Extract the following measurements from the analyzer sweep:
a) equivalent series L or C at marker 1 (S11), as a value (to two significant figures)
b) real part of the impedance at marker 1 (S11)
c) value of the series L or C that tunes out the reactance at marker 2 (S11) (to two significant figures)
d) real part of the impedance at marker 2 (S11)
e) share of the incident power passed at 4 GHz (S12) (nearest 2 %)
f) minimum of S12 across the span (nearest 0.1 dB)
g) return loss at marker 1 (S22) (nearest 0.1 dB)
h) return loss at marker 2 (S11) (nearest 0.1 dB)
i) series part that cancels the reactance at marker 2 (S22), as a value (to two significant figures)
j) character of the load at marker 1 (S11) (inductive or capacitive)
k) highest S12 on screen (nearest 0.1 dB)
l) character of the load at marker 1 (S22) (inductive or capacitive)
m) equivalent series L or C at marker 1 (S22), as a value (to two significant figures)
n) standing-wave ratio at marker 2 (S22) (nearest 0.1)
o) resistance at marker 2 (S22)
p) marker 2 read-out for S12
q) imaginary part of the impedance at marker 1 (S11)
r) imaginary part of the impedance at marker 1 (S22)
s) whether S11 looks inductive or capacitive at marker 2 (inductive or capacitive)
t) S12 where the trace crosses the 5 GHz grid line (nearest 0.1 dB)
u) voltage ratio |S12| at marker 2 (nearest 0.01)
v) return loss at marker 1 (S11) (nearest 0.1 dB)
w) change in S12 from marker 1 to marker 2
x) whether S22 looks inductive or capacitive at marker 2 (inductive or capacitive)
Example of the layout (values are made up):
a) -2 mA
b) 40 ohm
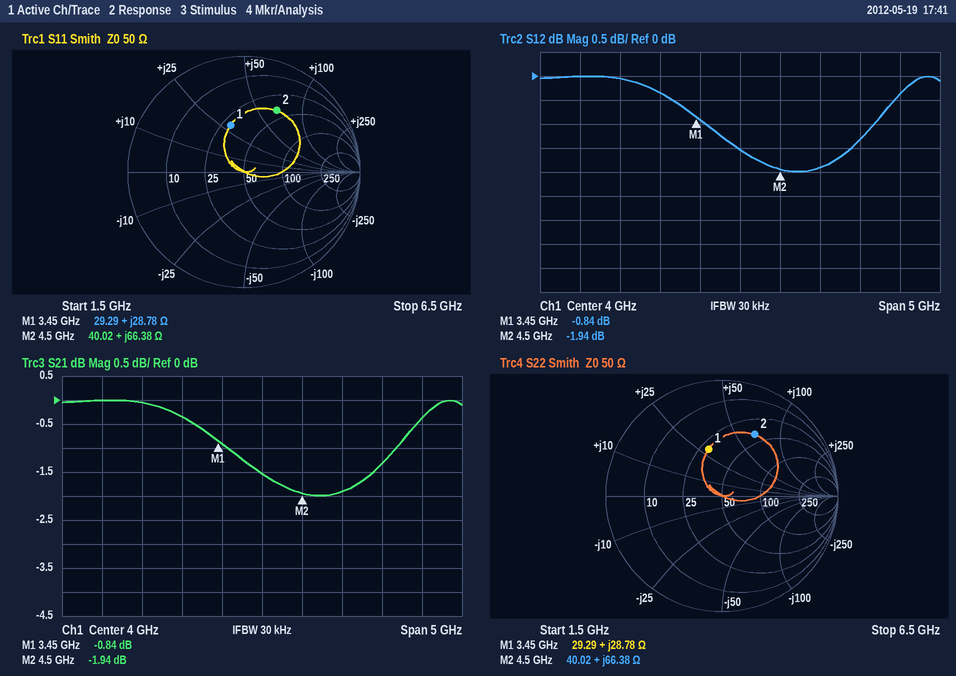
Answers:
a) 1.3 nH
b) 29.29 Ω
c) 530 fF
d) 40.02 Ω
e) 70 %
f) -2.0 dB
g) 7.5 dB
h) 4.4 dB
i) 530 fF
j) inductive
k) 0.0 dB
l) inductive
m) 1.3 nH
n) 4.0
o) 40.02 Ω
p) -1.94 dB
q) +28.78 Ω
r) +28.78 Ω
s) inductive
t) -1.9 dB
u) 0.80
v) 7.5 dB
w) -1.10 dB
x) inductive
